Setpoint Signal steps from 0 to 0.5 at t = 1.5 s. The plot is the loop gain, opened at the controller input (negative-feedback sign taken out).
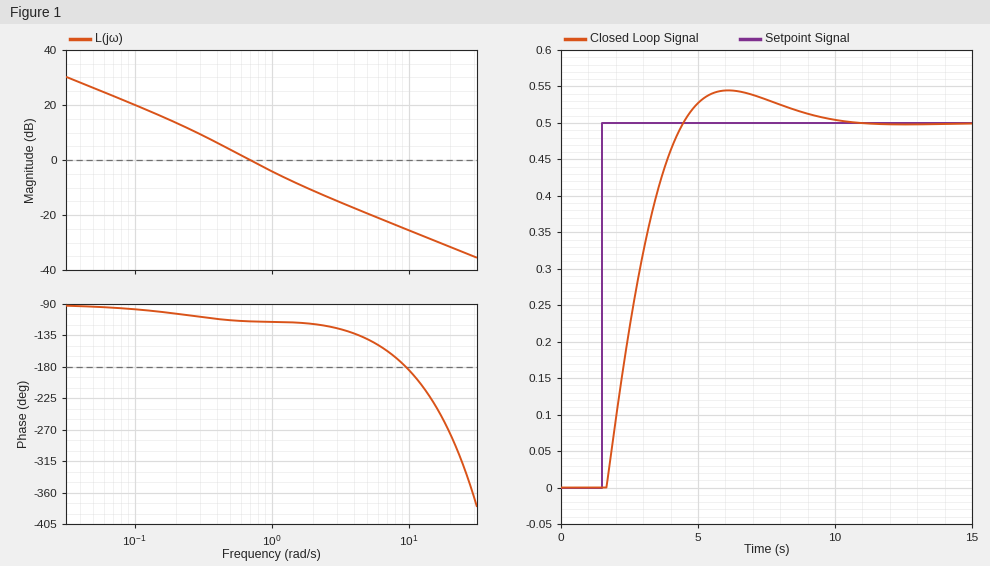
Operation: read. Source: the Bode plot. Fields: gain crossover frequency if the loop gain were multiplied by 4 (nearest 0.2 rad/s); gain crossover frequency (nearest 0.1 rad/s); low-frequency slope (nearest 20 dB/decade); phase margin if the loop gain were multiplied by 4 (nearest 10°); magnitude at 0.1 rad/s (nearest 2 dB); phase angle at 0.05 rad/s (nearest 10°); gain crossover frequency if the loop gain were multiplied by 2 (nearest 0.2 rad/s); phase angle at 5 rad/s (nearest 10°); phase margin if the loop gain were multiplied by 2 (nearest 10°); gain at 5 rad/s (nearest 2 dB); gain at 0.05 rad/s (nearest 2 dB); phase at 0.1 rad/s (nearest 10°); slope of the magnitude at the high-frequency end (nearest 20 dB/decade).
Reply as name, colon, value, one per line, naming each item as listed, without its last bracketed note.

gain crossover frequency if the loop gain were multiplied by 4: 2.2 rad/s
gain crossover frequency: 0.7 rad/s
low-frequency slope: -20 dB/decade
phase margin if the loop gain were multiplied by 4: 60°
magnitude at 0.1 rad/s: 20 dB
phase angle at 0.05 rad/s: -90°
gain crossover frequency if the loop gain were multiplied by 2: 1.2 rad/s
phase angle at 5 rad/s: -140°
phase margin if the loop gain were multiplied by 2: 60°
gain at 5 rad/s: -20 dB
gain at 0.05 rad/s: 26 dB
phase at 0.1 rad/s: -100°
slope of the magnitude at the high-frequency end: -20 dB/decade
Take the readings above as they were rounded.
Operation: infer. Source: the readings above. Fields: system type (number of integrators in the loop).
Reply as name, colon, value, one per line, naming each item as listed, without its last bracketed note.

system type: 1
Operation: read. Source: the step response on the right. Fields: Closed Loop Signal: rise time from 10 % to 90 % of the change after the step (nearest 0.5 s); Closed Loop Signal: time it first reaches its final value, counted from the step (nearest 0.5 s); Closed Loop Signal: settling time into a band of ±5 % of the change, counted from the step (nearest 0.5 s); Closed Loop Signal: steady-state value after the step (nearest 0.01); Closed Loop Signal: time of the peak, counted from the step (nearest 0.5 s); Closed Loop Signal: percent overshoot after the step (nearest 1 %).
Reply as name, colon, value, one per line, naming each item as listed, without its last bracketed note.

Closed Loop Signal: rise time from 10 % to 90 % of the change after the step: 2.0 s
Closed Loop Signal: time it first reaches its final value, counted from the step: 3.0 s
Closed Loop Signal: settling time into a band of ±5 % of the change, counted from the step: 6.5 s
Closed Loop Signal: steady-state value after the step: 0.50
Closed Loop Signal: time of the peak, counted from the step: 4.5 s
Closed Loop Signal: percent overshoot after the step: 9 %
